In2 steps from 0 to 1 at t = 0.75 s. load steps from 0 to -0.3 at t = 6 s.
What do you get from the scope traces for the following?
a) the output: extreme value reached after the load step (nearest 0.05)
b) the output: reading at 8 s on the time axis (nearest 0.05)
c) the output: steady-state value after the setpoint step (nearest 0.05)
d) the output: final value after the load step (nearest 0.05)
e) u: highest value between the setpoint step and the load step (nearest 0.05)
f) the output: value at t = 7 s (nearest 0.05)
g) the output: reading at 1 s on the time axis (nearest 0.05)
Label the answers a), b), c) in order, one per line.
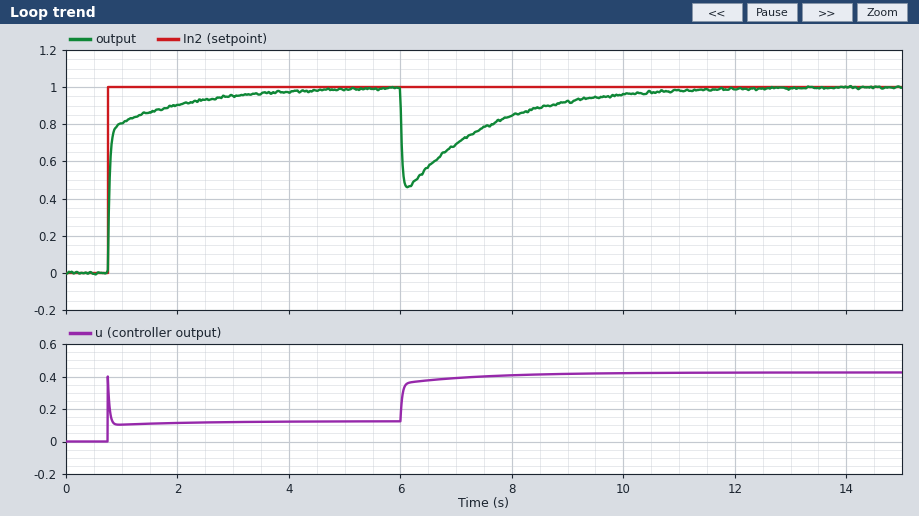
a) 0.45
b) 0.85
c) 1.00
d) 1.00
e) 0.40
f) 0.70
g) 0.80
